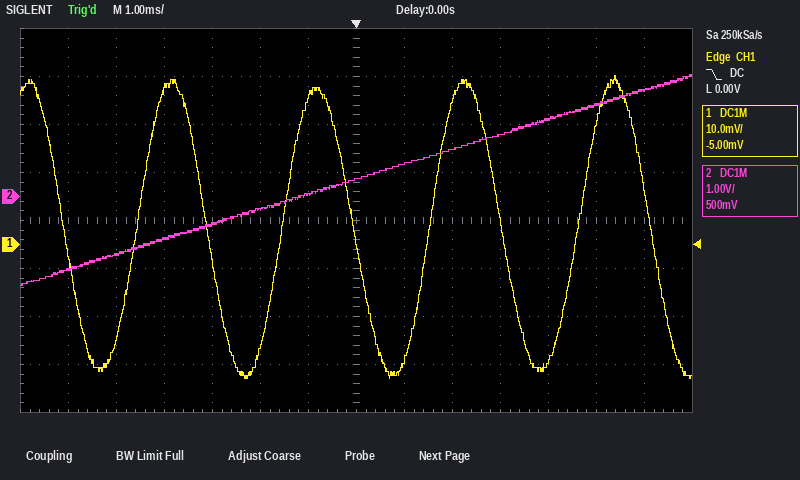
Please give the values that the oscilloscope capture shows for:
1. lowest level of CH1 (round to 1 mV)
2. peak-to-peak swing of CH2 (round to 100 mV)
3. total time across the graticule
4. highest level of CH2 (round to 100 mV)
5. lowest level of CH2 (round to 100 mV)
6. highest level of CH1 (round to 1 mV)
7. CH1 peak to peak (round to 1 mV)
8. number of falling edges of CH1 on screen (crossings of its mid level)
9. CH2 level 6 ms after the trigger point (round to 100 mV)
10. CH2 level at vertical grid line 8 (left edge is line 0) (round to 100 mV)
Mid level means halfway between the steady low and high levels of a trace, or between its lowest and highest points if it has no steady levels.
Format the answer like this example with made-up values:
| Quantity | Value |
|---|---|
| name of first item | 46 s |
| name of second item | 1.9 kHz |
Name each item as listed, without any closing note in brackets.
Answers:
| Quantity | Value |
|---|---|
| lowest level of CH1 | -28 mV |
| peak-to-peak swing of CH2 | 4.4 V |
| total time across the graticule | 14 ms |
| highest level of CH2 | 2.5 V |
| lowest level of CH2 | -1.9 V |
| highest level of CH1 | 35 mV |
| CH1 peak to peak | 63 mV |
| number of falling edges of CH1 on screen | 5 |
| CH2 level 6 ms after the trigger point | 2.2 V |
| CH2 level at vertical grid line 8 (left edge is line 0) | 700 mV |
